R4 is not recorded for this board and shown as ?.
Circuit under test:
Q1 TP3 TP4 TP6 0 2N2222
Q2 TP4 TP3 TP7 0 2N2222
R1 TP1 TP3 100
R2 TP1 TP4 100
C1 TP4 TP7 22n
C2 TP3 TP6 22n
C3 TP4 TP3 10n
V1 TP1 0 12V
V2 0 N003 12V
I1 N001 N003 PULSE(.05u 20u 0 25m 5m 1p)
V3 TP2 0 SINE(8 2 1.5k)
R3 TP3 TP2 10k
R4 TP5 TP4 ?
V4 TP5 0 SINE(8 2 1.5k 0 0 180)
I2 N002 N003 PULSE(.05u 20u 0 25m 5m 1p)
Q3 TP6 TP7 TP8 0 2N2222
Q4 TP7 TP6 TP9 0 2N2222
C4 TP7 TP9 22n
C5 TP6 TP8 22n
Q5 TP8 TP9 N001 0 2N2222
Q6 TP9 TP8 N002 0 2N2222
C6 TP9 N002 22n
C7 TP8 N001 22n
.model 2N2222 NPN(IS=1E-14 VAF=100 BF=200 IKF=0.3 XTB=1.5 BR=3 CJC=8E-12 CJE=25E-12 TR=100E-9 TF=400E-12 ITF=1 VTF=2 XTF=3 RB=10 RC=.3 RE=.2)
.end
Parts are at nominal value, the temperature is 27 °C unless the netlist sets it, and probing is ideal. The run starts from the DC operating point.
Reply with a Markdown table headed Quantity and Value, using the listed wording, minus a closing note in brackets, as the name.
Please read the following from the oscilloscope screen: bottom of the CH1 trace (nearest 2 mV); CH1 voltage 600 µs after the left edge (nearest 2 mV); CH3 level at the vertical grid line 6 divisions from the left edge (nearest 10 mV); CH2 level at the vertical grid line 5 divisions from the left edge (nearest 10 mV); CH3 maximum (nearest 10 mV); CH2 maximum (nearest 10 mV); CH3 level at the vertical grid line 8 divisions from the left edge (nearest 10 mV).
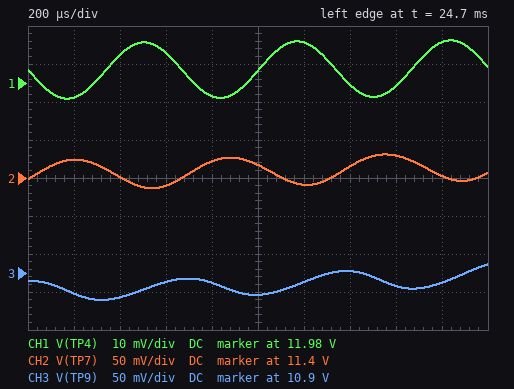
| Quantity | Value |
|---|---|
| bottom of the CH1 trace | 11.976 V |
| CH1 voltage 600 µs after the left edge | 11.988 V |
| CH3 level at the vertical grid line 6 divisions from the left edge | 10.89 V |
| CH2 level at the vertical grid line 5 divisions from the left edge | 11.42 V |
| CH3 maximum | 10.91 V |
| CH2 maximum | 11.43 V |
| CH3 level at the vertical grid line 8 divisions from the left edge | 10.88 V |
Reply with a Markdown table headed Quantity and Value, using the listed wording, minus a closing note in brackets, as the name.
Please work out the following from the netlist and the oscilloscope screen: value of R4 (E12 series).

| Quantity | Value |
|---|---|
| value of R4 | 27 kΩ |
